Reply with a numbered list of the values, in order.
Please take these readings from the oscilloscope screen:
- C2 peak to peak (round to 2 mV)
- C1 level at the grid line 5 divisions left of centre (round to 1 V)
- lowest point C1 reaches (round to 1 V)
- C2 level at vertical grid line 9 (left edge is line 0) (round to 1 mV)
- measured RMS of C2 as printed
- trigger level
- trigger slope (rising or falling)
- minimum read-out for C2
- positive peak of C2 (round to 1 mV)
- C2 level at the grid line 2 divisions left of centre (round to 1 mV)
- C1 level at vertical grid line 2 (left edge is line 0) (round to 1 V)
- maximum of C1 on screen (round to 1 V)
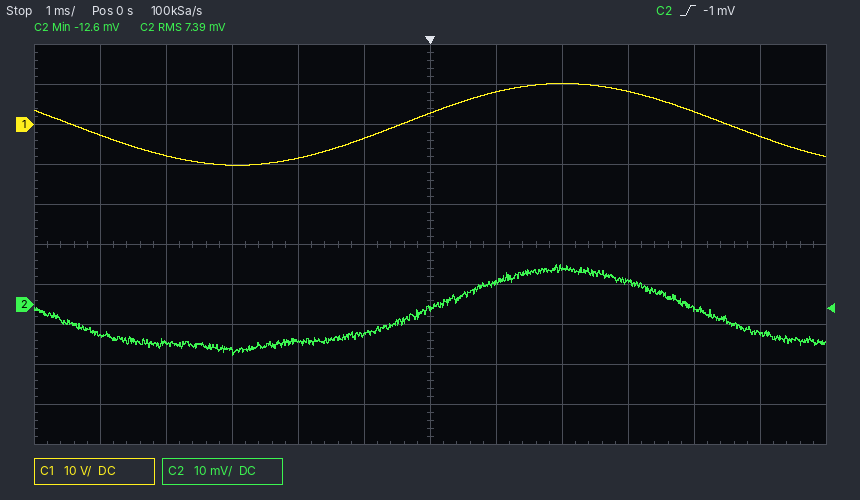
1. 22 mV
2. -3 V
3. -10 V
4. 6 mV
5. 7.39 mV
6. -1 mV
7. rising
8. -12.6 mV
9. 10 mV
10. -9 mV
11. -8 V
12. 10 V
